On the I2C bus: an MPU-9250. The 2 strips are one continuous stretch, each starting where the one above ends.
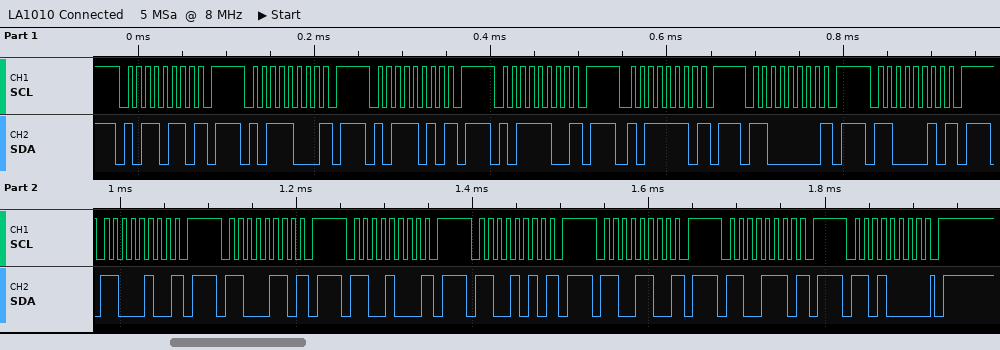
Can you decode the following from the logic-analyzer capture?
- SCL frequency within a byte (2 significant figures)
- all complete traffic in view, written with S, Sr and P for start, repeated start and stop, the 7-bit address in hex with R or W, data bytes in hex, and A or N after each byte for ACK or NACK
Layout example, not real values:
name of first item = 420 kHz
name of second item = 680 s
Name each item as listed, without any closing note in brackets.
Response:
SCL frequency within a byte = 100 kHz
all complete traffic in view, written with S, Sr and P for start, repeated start and stop, the 7-bit address in hex with R or W, data bytes in hex, and A or N after each byte for ACK or NACK = S 5BW N P S 5CW N P S 5DW N P S 5EW N P S 5FW N P S 60W N P S 61W N P S 62W N P S 63W N P S 64W N P S 65W N P S 66W N P S 67W N P S 68W A P
